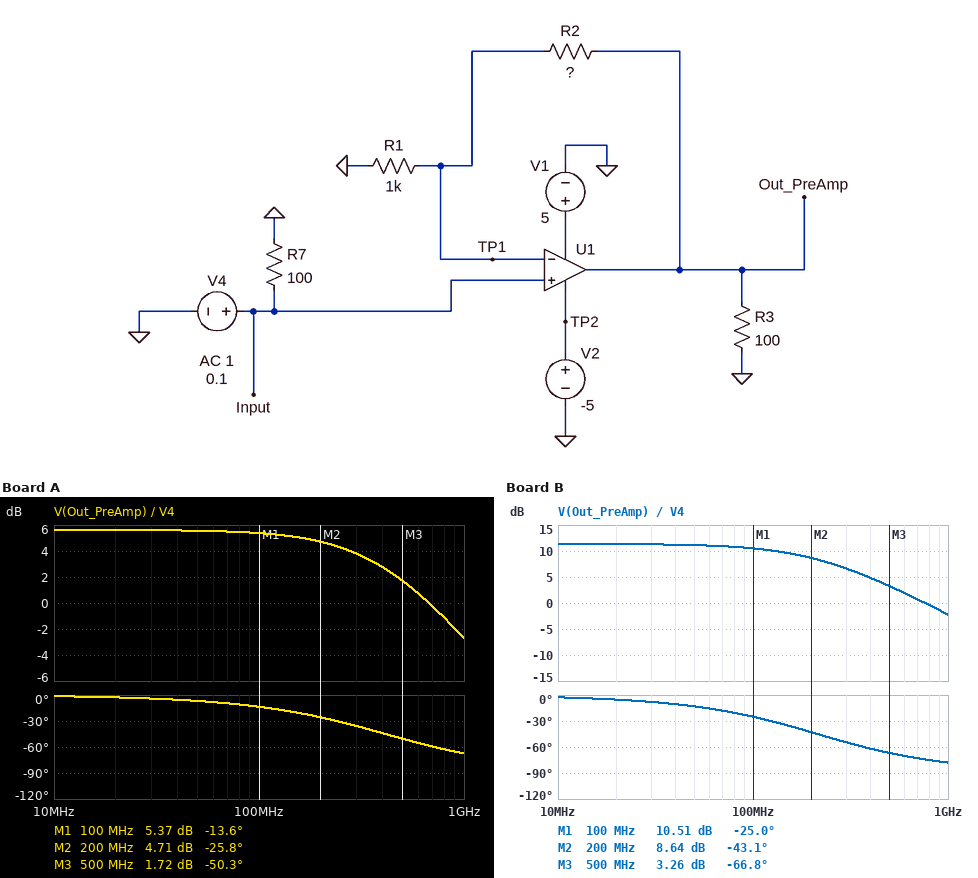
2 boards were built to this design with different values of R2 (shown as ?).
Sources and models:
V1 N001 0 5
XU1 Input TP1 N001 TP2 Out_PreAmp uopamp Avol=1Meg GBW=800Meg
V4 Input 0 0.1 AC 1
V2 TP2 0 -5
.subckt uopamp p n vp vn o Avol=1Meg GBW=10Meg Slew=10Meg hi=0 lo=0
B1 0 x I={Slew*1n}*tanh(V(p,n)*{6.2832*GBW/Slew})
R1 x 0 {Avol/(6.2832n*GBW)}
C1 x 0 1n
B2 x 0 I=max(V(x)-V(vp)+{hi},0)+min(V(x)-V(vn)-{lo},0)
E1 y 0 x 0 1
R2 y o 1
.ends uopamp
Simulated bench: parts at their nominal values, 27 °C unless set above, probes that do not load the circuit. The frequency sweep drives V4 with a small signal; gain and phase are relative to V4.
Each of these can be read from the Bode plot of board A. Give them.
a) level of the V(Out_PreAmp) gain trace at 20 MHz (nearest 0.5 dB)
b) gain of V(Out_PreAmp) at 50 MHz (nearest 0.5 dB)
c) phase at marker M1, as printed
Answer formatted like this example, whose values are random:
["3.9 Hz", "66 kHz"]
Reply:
["5.5 dB", "5.5 dB", "-13.6 deg"]
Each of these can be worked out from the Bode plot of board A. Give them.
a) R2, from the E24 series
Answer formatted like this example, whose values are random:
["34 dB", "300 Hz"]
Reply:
["910 Ω"]
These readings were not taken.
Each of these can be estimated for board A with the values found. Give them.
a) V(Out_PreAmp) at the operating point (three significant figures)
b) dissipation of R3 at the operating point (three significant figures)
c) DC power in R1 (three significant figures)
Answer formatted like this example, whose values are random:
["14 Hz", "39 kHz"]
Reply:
["191 mV", "365 µW", "10.0 µW"]
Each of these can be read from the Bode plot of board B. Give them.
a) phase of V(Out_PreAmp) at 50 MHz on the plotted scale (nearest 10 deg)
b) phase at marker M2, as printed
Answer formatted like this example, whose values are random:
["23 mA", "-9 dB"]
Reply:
["-10 deg", "-43.1 deg"]
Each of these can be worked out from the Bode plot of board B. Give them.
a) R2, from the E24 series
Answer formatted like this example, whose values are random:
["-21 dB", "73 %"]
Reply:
["2.7 kΩ"]
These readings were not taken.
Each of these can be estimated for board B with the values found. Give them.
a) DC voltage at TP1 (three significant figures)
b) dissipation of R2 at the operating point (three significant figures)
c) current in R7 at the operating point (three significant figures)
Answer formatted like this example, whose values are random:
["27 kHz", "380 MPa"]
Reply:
["100 mV", "27.0 µW", "1.00 mA"]
